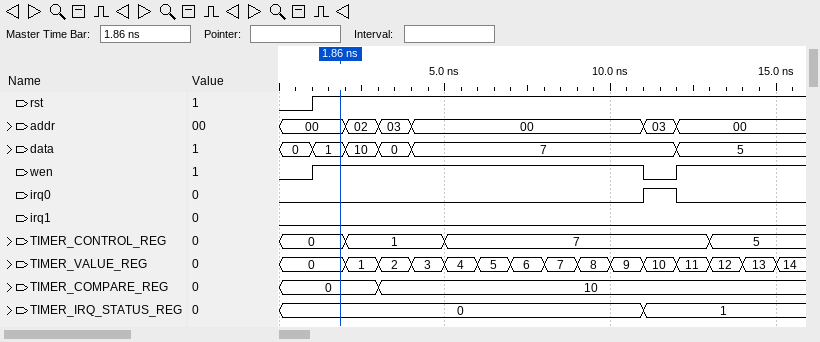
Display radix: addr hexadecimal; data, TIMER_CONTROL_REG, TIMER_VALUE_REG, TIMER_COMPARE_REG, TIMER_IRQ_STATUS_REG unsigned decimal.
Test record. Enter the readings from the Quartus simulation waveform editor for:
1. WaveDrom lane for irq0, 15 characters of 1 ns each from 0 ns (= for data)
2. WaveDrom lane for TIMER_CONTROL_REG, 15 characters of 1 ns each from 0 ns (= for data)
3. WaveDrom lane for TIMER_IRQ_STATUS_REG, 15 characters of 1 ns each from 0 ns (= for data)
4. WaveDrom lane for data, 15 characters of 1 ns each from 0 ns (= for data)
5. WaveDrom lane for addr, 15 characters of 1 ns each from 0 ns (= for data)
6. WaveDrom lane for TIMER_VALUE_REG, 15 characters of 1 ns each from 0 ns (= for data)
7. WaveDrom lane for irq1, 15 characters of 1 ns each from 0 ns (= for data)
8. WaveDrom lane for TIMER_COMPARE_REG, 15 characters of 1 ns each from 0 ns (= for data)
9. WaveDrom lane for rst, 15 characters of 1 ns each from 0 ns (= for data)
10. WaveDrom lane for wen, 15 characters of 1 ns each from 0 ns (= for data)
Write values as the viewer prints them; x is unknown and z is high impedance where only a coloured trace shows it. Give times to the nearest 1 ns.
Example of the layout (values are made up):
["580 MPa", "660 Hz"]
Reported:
["{name: 'irq0', wave: '0..........10..'}", "{name: 'TIMER_CONTROL_REG', wave: '=.=..=.......=.', data: '0 1 7 5'}", "{name: 'TIMER_IRQ_STATUS_REG', wave: '=..........=...', data: '0 1'}", "{name: 'data', wave: '=====.......=..', data: '0 1 10 0 7 5'}", "{name: 'addr', wave: '=.===......==..', data: '00 02 03 00 03 00'}", "{name: 'TIMER_VALUE_REG', wave: '=.=============', data: '0 1 2 3 4 5 6 7 8 9 10 11 12 13'}", "{name: 'irq1', wave: '0..............'}", "{name: 'TIMER_COMPARE_REG', wave: '=..=...........', data: '0 10'}", "{name: 'rst', wave: '01.............'}", "{name: 'wen', wave: '01.........01..'}"]
